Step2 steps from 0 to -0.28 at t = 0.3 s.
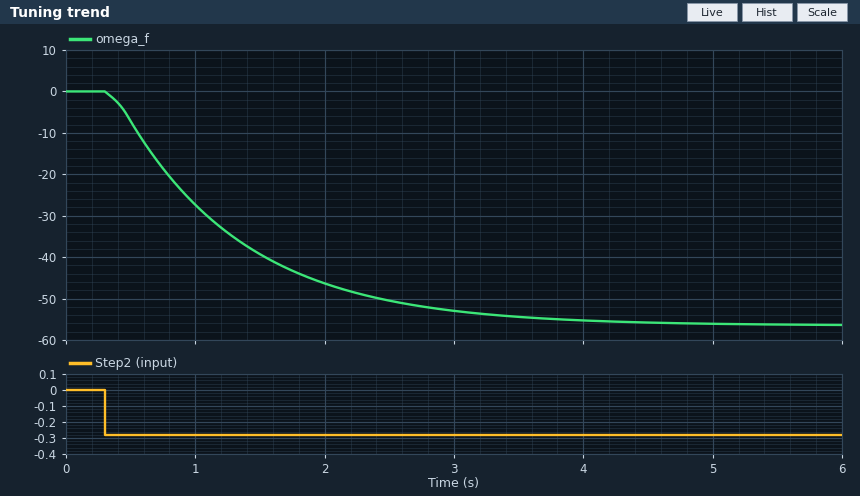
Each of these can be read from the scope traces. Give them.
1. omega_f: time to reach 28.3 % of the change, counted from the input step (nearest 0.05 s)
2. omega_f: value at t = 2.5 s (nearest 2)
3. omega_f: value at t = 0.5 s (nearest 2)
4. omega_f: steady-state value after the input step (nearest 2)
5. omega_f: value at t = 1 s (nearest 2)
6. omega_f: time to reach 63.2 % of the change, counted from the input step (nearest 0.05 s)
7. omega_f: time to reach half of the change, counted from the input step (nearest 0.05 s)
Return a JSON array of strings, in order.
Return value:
["0.40 s", "-50", "-8", "-56", "-28", "1.00 s", "0.75 s"]
